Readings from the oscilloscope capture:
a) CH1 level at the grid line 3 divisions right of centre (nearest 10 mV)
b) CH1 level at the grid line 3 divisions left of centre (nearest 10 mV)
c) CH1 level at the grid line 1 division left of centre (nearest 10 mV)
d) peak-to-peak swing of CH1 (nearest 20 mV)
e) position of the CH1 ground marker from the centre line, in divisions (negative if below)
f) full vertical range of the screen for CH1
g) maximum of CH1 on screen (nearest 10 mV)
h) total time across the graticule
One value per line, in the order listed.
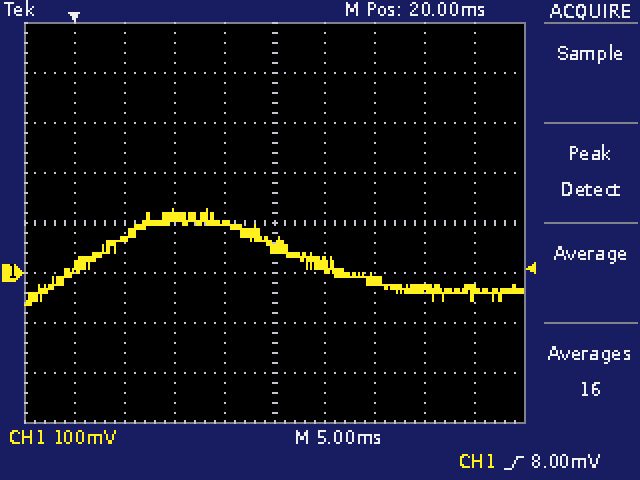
-30 mV
70 mV
100 mV
200 mV
-1.0 div
800 mV
130 mV
50 ms
